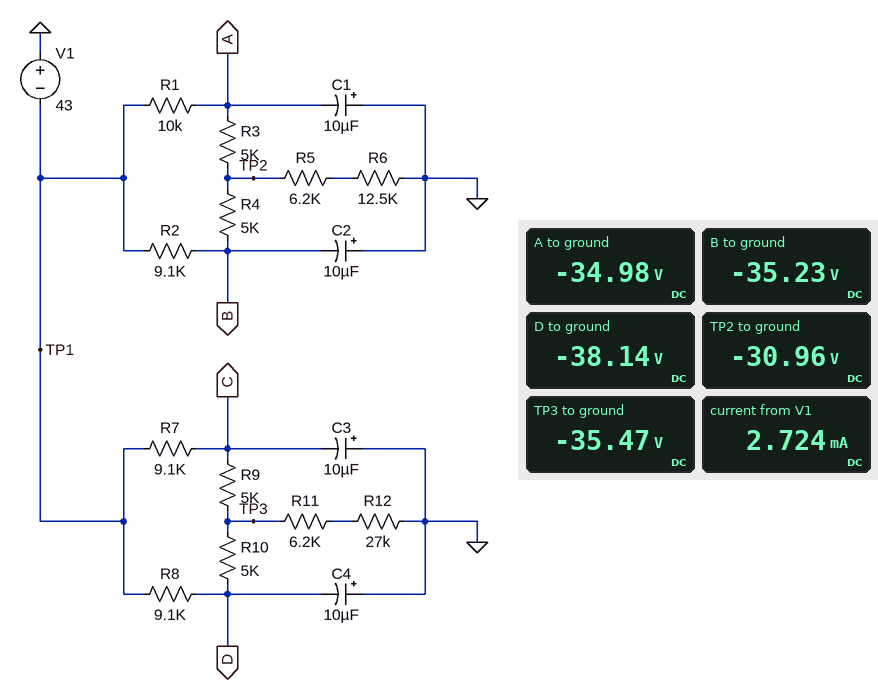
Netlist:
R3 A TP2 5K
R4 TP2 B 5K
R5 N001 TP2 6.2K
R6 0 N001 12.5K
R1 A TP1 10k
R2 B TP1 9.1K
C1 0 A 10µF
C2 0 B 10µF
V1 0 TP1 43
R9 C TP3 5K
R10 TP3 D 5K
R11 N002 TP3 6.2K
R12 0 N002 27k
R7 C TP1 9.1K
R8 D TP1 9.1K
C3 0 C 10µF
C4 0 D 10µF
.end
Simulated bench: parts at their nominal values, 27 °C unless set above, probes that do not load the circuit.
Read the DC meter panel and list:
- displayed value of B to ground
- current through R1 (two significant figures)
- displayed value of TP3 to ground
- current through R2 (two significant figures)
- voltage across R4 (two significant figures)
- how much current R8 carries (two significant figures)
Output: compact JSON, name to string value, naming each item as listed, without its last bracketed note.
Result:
{"displayed value of B to ground": "-35.23 V", "current through R1": "800 µA", "displayed value of TP3 to ground": "-35.47 V", "current through R2": "850 µA", "voltage across R4": "4.3 V", "how much current R8 carries": "530 µA"}
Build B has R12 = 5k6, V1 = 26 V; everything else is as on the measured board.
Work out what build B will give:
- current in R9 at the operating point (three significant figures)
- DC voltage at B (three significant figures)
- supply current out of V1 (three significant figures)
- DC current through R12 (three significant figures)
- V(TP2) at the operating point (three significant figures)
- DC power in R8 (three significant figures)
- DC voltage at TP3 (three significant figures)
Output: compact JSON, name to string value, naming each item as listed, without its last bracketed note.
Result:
{"current in R9 at the operating point": "690 µA", "DC voltage at B": "-21.3 V", "supply current out of V1": "2.38 mA", "DC current through R12": "1.38 mA", "V(TP2) at the operating point": "-18.7 V", "DC power in R8": "4.33 mW", "DC voltage at TP3": "-16.3 V"}
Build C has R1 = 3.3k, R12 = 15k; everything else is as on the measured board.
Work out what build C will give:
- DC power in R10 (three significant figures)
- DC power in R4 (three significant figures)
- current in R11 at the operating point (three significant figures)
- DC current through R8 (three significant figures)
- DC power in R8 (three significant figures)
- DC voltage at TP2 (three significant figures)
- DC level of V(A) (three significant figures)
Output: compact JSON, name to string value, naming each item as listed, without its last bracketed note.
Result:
{"DC power in R10": "2.90 mW", "DC power in R4": "2.22 mW", "current in R11 at the operating point": "1.52 mA", "DC current through R8": "761 µA", "DC power in R8": "5.27 mW", "DC voltage at TP2": "-33.6 V", "DC level of V(A)": "-39.3 V"}
